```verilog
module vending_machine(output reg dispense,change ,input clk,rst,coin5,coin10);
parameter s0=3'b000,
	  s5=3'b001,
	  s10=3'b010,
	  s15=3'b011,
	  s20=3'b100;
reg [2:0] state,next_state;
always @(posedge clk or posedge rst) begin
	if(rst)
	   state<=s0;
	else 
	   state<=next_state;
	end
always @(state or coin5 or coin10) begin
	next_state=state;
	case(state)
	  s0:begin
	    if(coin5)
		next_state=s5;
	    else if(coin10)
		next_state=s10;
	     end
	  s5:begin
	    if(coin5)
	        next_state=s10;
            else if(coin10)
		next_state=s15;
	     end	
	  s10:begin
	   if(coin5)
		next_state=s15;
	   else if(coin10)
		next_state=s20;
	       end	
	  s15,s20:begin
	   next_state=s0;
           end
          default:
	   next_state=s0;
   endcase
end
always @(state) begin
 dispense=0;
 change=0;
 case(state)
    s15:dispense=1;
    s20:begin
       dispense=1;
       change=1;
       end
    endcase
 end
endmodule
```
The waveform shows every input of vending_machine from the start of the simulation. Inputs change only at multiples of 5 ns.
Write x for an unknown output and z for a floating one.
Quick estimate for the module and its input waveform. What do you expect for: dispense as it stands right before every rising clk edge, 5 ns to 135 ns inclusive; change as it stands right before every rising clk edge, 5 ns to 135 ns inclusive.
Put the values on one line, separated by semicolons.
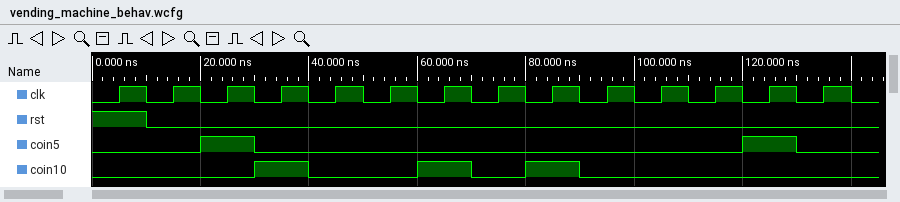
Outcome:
0 0 0 0 1 0 0 0 0 1 0 0 0 0; 0 0 0 0 0 0 0 0 0 1 0 0 0 0
